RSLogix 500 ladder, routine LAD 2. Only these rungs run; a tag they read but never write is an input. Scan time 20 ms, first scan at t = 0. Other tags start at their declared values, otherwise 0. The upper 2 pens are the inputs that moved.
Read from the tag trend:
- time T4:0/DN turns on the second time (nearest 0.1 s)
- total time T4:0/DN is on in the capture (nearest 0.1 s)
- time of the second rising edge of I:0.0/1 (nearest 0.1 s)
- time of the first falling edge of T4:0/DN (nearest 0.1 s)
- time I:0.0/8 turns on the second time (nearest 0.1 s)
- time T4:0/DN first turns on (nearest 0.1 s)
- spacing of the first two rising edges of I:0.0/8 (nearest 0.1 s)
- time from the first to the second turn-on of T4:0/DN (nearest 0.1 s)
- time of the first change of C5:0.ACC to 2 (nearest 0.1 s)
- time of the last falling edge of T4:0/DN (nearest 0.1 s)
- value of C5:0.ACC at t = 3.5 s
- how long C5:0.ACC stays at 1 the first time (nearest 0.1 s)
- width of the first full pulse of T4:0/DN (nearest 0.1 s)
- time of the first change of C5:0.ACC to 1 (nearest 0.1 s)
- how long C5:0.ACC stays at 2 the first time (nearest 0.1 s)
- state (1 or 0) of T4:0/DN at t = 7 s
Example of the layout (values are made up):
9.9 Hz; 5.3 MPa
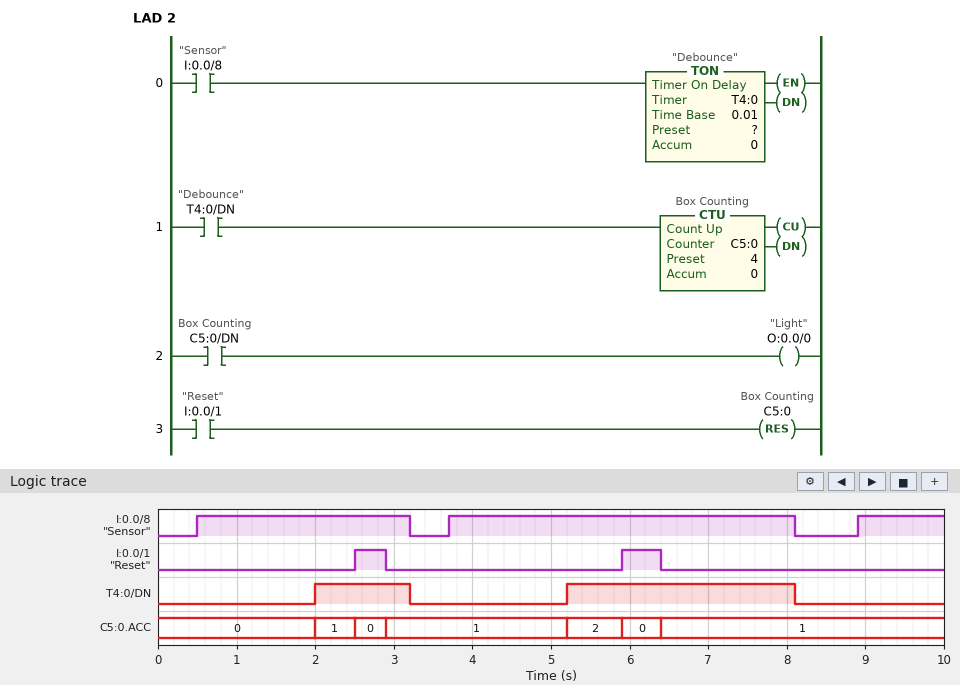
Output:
5.2 s; 4.1 s; 5.9 s; 3.2 s; 3.7 s; 2.0 s; 3.2 s; 3.2 s; 5.2 s; 8.1 s; 1; 0.5 s; 1.2 s; 2.0 s; 0.7 s; 1
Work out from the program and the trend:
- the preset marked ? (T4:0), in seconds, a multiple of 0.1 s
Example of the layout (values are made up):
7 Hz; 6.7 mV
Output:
1.5 s
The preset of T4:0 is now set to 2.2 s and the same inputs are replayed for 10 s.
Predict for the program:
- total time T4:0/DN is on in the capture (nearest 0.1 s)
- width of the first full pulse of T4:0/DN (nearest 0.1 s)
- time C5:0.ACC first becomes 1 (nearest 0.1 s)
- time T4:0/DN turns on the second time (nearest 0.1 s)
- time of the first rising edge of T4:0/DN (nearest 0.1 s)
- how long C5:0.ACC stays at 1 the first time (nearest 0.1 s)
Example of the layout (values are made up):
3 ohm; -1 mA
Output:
2.7 s; 0.5 s; 2.9 s; 5.9 s; 2.7 s; 3.0 s
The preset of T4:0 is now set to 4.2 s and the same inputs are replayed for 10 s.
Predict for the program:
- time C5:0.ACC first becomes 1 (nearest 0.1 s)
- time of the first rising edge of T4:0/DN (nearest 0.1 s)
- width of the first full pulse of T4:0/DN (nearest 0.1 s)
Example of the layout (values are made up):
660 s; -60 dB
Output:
7.9 s; 7.9 s; 0.2 s
